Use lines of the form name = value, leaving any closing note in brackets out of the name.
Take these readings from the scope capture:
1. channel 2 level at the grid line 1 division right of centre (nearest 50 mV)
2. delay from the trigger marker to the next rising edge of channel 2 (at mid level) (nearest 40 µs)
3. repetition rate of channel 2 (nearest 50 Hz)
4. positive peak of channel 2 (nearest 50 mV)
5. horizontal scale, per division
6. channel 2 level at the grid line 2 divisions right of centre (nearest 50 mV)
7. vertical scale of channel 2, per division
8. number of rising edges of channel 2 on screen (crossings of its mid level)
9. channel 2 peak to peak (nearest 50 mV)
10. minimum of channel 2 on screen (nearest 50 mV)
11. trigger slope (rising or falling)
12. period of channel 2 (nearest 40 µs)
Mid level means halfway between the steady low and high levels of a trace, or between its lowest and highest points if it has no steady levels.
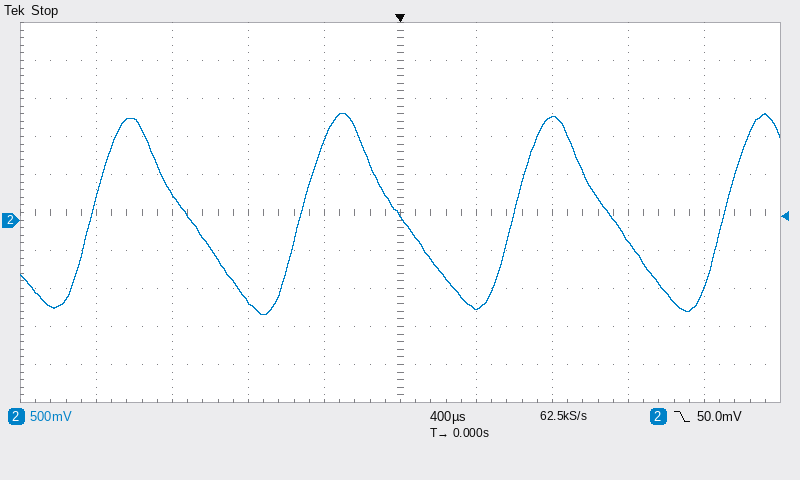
channel 2 level at the grid line 1 division right of centre = -1.15 V
delay from the trigger marker to the next rising edge of channel 2 (at mid level) = 600 µs
repetition rate of channel 2 = 900 Hz
positive peak of channel 2 = 1.40 V
horizontal scale, per division = 400 µs
channel 2 level at the grid line 2 divisions right of centre = 1.35 V
vertical scale of channel 2, per division = 500 mV
number of rising edges of channel 2 on screen = 4
channel 2 peak to peak = 2.65 V
minimum of channel 2 on screen = -1.25 V
trigger slope = falling
period of channel 2 = 1.12 ms
